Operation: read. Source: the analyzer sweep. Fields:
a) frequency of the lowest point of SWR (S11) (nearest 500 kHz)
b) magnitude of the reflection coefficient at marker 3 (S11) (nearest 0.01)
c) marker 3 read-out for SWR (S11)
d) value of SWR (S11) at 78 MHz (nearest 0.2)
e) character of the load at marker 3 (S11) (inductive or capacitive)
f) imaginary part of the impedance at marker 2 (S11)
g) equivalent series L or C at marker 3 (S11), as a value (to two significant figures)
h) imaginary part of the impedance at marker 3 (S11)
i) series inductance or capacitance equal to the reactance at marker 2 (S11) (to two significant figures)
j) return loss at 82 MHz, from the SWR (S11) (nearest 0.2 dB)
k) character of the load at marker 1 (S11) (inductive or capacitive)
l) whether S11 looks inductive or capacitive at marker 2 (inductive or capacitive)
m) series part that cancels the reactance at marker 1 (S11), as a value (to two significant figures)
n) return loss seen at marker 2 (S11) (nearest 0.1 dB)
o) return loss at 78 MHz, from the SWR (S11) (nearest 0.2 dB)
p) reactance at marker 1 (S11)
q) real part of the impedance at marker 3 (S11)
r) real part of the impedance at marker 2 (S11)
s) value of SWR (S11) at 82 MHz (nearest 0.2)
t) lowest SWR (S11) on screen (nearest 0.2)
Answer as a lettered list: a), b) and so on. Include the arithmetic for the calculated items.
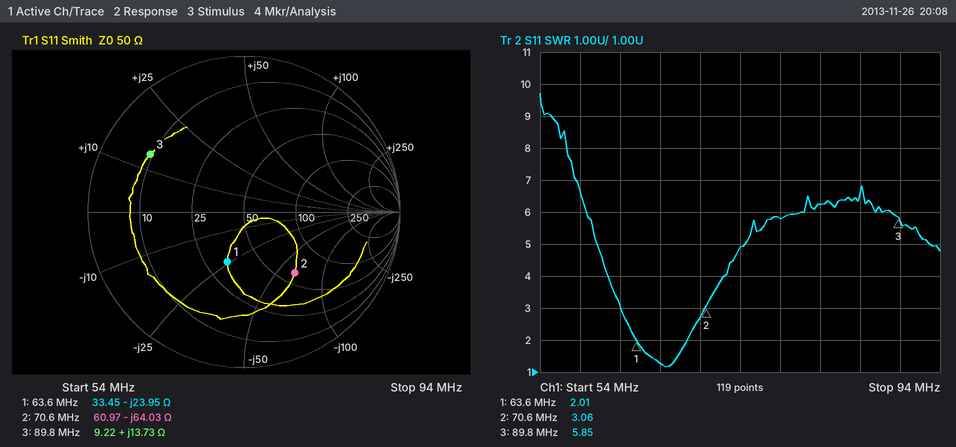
a) 66.5 MHz
b) 0.71
c) 5.85
d) 5.8
e) inductive
f) -64.03 Ω
g) L = 13.73 Ω/(2π × 89.8 MHz) ≈ 24 nH
h) +13.73 Ω
i) C = 1/(2π × 70.6 MHz × 64.03 Ω) ≈ 35 pF
j) −20 log10((6.2 − 1)/(6.2 + 1)) ≈ 2.8 dB
k) capacitive
l) capacitive
m) L = 23.95 Ω/(2π × 63.6 MHz) ≈ 60 nH
n) 5.9 dB
o) −20 log10((5.8 − 1)/(5.8 + 1)) ≈ 3.0 dB
p) -23.95 Ω
q) 9.22 Ω
r) 60.97 Ω
s) 6.2
t) 1.2
